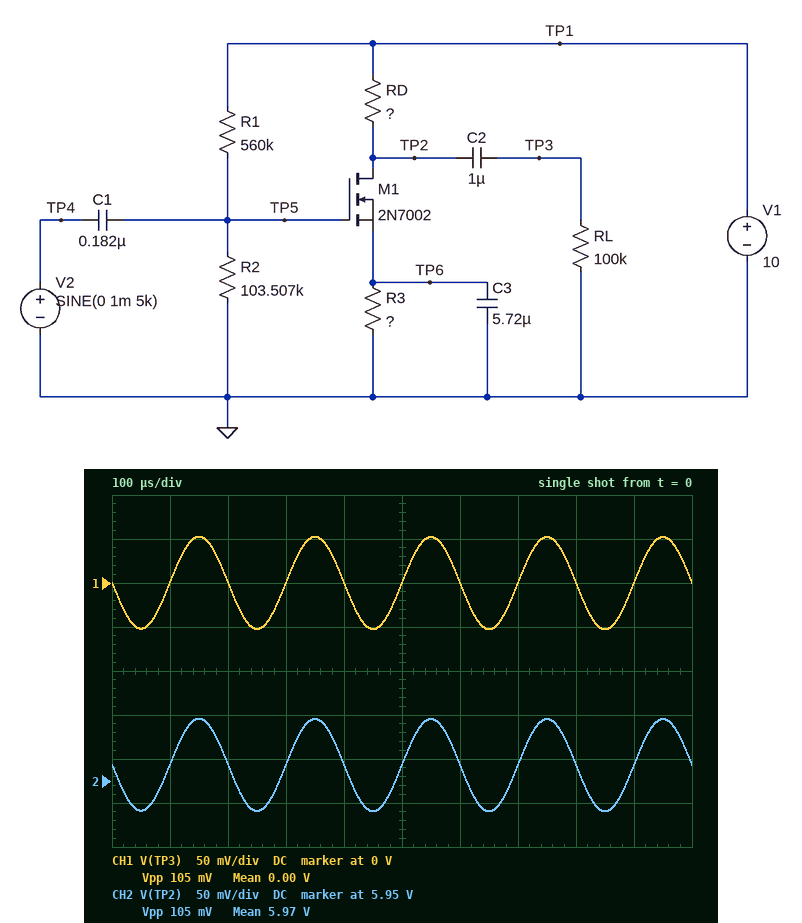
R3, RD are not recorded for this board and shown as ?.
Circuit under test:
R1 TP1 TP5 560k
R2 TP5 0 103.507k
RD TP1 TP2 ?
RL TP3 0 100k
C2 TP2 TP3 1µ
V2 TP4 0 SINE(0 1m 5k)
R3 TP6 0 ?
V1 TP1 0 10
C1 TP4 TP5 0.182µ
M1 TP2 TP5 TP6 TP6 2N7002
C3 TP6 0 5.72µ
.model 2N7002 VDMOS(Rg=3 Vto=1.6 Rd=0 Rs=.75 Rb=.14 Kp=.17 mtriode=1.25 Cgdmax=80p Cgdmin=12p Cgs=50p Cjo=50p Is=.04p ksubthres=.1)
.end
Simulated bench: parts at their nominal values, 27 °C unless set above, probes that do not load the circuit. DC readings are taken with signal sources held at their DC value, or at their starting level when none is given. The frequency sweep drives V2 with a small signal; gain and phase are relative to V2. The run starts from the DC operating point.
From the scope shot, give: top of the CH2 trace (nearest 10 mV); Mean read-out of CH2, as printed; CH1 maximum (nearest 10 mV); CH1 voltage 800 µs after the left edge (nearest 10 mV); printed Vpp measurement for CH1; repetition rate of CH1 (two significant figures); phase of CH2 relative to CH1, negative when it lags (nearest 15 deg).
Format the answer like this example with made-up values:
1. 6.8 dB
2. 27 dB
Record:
1. 6.02 V
2. 5.97 V
3. 50 mV
4. 0 V
5. 105 mV
6. 5.0 kHz
7. 0 deg
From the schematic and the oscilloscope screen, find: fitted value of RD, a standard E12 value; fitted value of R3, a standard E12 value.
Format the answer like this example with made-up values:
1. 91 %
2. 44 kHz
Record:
1. 22 kΩ
2. 68 Ω
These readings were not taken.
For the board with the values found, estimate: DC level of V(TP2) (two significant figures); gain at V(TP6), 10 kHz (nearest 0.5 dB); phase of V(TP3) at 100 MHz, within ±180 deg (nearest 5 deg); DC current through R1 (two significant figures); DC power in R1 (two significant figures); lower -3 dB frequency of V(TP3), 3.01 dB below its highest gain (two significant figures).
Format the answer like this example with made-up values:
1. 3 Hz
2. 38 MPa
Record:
1. 6.0 V
2. -42.0 dB
3. 10 deg
4. 15 µA
5. 130 µW
6. 16 Hz
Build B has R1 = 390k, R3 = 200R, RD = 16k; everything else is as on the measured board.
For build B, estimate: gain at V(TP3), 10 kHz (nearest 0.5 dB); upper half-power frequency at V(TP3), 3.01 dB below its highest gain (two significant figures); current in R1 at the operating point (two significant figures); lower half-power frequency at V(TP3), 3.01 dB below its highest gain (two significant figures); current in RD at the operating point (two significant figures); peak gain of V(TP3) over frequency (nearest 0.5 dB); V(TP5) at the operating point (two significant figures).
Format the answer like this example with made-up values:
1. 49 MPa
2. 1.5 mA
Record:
1. -33.5 dB
2. 850 MHz
3. 20 µA
4. 67 MHz
5. 620 µA
6. -6.0 dB
7. 2.1 V
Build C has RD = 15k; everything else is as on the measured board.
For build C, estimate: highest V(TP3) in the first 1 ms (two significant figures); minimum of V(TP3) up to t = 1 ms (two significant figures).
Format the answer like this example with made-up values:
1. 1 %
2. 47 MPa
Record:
1. 38 mV
2. -38 mV
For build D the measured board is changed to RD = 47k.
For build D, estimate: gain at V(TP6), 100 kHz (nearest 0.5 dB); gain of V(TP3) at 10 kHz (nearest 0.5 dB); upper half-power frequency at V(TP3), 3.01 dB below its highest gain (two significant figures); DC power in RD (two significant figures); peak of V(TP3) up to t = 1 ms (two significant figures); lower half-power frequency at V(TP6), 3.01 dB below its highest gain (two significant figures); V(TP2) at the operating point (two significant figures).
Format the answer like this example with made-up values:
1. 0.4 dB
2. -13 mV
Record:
1. -64.5 dB
2. 39.0 dB
3. 58 kHz
4. 1.6 mW
5. 91 mV
6. 9.4 Hz
7. 1.4 V
